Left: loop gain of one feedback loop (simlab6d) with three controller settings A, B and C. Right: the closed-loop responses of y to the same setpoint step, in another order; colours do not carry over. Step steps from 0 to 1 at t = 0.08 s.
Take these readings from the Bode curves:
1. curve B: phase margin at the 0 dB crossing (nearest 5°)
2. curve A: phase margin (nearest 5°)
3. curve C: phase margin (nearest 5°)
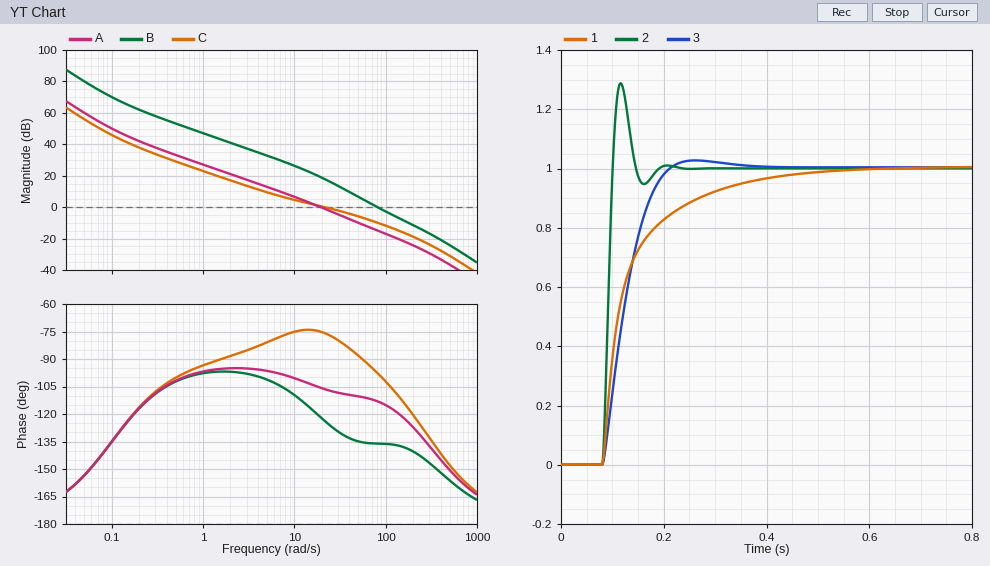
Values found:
45°
75°
105°
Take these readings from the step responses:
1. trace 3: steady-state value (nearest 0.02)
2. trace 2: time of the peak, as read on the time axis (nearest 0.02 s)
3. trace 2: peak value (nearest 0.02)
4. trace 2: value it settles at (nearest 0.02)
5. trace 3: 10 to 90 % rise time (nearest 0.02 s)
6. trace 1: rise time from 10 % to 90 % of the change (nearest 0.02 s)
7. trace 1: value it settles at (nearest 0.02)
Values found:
1.00
0.12 s
1.28
1.00
0.08 s
0.18 s
1.00
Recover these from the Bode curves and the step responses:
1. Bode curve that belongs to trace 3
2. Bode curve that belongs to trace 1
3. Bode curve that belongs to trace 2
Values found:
A
C
B
